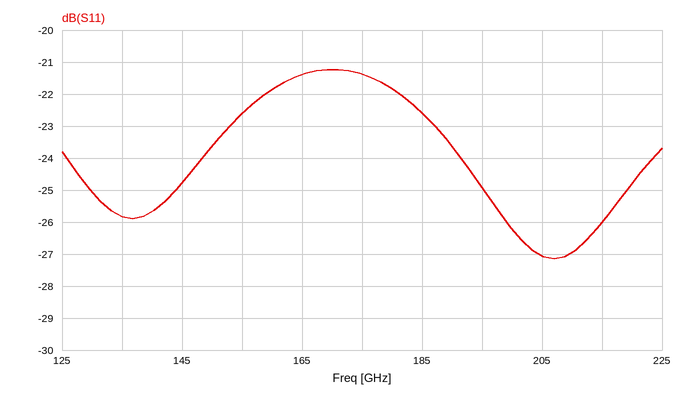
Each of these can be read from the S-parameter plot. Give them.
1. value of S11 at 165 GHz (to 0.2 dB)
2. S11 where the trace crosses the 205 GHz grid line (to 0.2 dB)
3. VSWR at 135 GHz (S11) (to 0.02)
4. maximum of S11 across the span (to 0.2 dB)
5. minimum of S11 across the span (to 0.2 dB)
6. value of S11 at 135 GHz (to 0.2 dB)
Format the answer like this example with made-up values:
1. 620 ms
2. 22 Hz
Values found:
1. -21.4 dB
2. -27.0 dB
3. 1.10
4. -21.2 dB
5. -27.2 dB
6. -25.8 dB
